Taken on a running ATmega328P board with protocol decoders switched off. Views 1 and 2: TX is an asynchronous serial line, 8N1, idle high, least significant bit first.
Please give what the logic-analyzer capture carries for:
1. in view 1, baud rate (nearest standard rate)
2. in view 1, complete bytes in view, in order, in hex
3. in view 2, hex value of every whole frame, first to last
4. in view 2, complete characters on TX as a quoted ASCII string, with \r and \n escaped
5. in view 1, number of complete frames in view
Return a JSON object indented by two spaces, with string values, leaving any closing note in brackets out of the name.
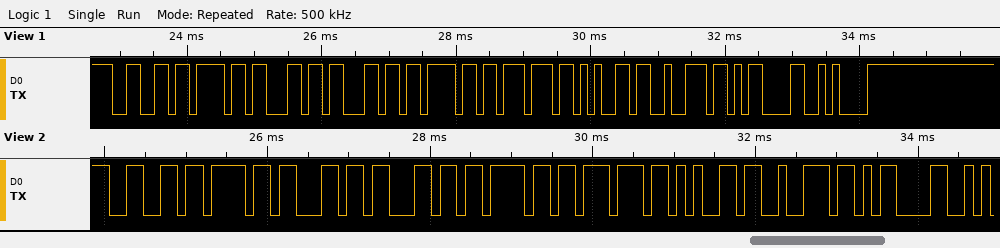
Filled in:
{
  "in view 1, baud rate": "9600 baud",
  "in view 1, complete bytes in view, in order, in hex": "0x66 0x6F 0x6C 0x6C 0x6F 0x77 0x65 0x72 0x0D 0x0A",
  "in view 2, hex value of every whole frame, first to last": "66 6F 6C 6C 6F 77 65 72 0D",
  "in view 2, complete characters on TX as a quoted ASCII string, with \\r and \\n escaped": "\"follower\\r\"",
  "in view 1, number of complete frames in view": "10"
}
